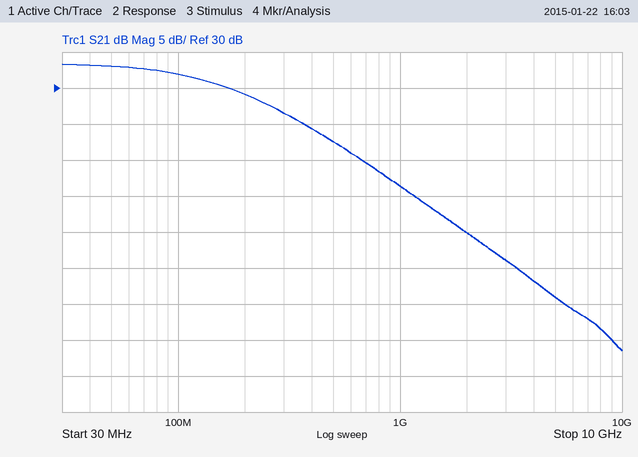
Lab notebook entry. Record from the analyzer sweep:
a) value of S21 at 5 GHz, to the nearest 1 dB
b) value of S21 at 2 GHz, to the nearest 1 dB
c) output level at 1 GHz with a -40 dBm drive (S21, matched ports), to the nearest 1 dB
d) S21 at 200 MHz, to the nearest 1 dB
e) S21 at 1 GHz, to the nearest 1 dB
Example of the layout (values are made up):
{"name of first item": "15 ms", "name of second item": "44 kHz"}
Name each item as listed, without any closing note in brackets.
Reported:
{"value of S21 at 5 GHz, to the nearest 1 dB": "1 dB", "value of S21 at 2 GHz, to the nearest 1 dB": "10 dB", "output level at 1 GHz with a -40 dBm drive (S21, matched ports), to the nearest 1 dB": "-24 dBm", "S21 at 200 MHz, to the nearest 1 dB": "29 dB", "S21 at 1 GHz, to the nearest 1 dB": "16 dB"}
